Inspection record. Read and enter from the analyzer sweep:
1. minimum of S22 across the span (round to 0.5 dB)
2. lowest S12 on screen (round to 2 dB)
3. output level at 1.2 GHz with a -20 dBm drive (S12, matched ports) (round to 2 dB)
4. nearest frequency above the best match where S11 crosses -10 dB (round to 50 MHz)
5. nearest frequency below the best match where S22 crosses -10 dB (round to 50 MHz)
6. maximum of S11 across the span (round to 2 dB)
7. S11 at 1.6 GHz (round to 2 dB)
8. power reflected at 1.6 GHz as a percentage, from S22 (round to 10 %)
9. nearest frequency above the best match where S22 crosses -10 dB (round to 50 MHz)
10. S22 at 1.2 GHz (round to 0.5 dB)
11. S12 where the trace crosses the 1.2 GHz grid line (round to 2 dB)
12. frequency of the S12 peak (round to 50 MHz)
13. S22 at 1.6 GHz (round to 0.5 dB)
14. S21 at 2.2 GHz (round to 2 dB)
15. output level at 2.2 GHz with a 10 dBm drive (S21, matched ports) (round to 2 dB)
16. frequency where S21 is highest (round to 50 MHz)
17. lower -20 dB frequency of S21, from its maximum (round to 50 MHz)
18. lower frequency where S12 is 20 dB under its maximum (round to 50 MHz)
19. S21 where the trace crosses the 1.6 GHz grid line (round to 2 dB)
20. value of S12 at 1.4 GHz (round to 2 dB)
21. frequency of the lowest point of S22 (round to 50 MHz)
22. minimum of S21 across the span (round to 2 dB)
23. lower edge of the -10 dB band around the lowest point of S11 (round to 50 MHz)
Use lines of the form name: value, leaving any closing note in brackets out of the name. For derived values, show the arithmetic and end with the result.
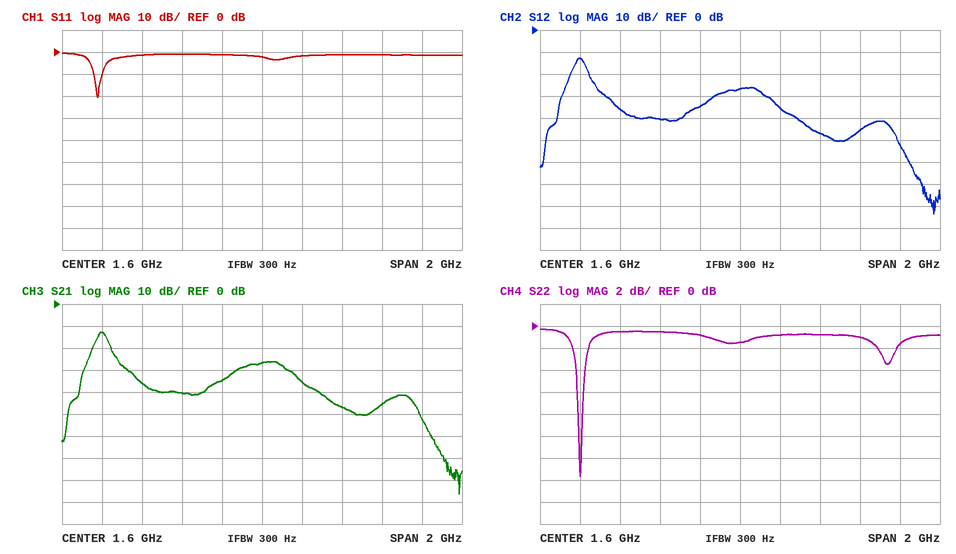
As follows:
minimum of S22 across the span: -13.5 dB
lowest S12 on screen: -84 dB
output level at 1.2 GHz with a -20 dBm drive (S12, matched ports): -20 dBm + (-40 dB) = -60 dBm
nearest frequency above the best match where S11 crosses -10 dB: 800 MHz
nearest frequency below the best match where S22 crosses -10 dB: 800 MHz
maximum of S11 across the span: 0 dB
S11 at 1.6 GHz: -2 dB
power reflected at 1.6 GHz as a percentage, from S22: 10^(-1.5/10) ≈ 70.8 %, so 70 % to the nearest 10 %
nearest frequency above the best match where S22 crosses -10 dB: 800 MHz
S22 at 1.2 GHz: -0.5 dB
S12 where the trace crosses the 1.2 GHz grid line: -40 dB
frequency of the S12 peak: 800 MHz
S22 at 1.6 GHz: -1.5 dB
S21 at 2.2 GHz: -46 dB
output level at 2.2 GHz with a 10 dBm drive (S21, matched ports): 10 dBm + (-46 dB) = -36 dBm
frequency where S21 is highest: 800 MHz
lower -20 dB frequency of S21, from its maximum: 700 MHz
lower frequency where S12 is 20 dB under its maximum: 700 MHz
S21 where the trace crosses the 1.6 GHz grid line: -26 dB
value of S12 at 1.4 GHz: -34 dB
frequency of the lowest point of S22: 800 MHz
minimum of S21 across the span: -86 dB
lower edge of the -10 dB band around the lowest point of S11: 750 MHz
